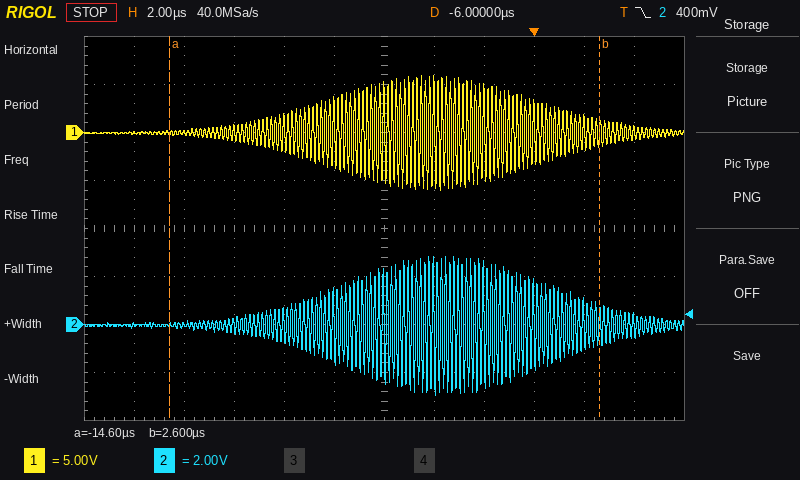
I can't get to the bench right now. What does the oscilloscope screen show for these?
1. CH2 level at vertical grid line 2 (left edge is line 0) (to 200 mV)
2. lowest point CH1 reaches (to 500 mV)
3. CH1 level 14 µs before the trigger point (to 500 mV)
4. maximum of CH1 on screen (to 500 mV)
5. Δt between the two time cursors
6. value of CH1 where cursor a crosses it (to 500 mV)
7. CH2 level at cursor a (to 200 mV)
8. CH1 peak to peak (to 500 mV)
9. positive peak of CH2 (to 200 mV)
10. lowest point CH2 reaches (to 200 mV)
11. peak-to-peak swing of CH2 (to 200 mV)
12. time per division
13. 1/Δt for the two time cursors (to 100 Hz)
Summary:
0.0 V
-6.0 V
0.0 V
6.0 V
17.2 µs
0.0 V
0.0 V
12.0 V
2.8 V
-3.0 V
5.8 V
2 µs
58.1 kHz
